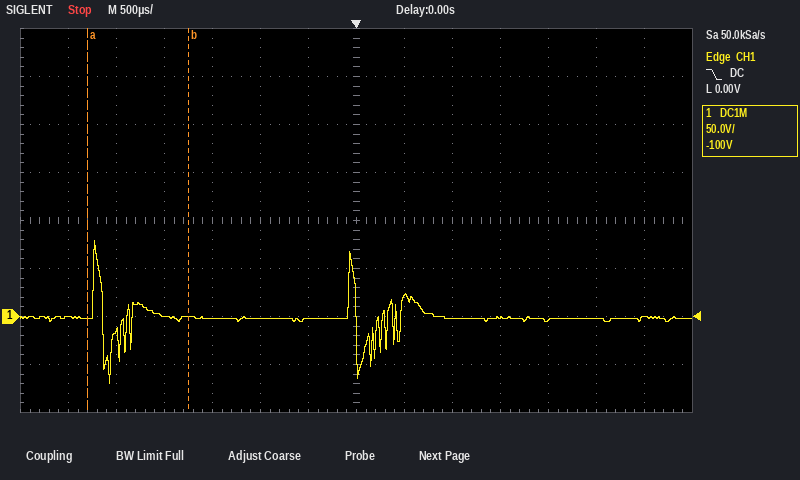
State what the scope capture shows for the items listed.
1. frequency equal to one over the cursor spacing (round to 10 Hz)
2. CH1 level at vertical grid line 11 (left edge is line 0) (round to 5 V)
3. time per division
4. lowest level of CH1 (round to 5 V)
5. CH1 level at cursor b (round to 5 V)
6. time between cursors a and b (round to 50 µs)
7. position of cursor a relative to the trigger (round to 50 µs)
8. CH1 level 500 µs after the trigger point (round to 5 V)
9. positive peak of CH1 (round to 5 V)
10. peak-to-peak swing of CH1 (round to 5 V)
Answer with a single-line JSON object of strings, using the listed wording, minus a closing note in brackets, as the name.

{"frequency equal to one over the cursor spacing": "950 Hz", "CH1 level at vertical grid line 11 (left edge is line 0)": "-5 V", "time per division": "500 µs", "lowest level of CH1": "-70 V", "CH1 level at cursor b": "0 V", "time between cursors a and b": "1.05 ms", "position of cursor a relative to the trigger": "-2.80 ms", "CH1 level 500 µs after the trigger point": "20 V", "positive peak of CH1": "80 V", "peak-to-peak swing of CH1": "150 V"}
